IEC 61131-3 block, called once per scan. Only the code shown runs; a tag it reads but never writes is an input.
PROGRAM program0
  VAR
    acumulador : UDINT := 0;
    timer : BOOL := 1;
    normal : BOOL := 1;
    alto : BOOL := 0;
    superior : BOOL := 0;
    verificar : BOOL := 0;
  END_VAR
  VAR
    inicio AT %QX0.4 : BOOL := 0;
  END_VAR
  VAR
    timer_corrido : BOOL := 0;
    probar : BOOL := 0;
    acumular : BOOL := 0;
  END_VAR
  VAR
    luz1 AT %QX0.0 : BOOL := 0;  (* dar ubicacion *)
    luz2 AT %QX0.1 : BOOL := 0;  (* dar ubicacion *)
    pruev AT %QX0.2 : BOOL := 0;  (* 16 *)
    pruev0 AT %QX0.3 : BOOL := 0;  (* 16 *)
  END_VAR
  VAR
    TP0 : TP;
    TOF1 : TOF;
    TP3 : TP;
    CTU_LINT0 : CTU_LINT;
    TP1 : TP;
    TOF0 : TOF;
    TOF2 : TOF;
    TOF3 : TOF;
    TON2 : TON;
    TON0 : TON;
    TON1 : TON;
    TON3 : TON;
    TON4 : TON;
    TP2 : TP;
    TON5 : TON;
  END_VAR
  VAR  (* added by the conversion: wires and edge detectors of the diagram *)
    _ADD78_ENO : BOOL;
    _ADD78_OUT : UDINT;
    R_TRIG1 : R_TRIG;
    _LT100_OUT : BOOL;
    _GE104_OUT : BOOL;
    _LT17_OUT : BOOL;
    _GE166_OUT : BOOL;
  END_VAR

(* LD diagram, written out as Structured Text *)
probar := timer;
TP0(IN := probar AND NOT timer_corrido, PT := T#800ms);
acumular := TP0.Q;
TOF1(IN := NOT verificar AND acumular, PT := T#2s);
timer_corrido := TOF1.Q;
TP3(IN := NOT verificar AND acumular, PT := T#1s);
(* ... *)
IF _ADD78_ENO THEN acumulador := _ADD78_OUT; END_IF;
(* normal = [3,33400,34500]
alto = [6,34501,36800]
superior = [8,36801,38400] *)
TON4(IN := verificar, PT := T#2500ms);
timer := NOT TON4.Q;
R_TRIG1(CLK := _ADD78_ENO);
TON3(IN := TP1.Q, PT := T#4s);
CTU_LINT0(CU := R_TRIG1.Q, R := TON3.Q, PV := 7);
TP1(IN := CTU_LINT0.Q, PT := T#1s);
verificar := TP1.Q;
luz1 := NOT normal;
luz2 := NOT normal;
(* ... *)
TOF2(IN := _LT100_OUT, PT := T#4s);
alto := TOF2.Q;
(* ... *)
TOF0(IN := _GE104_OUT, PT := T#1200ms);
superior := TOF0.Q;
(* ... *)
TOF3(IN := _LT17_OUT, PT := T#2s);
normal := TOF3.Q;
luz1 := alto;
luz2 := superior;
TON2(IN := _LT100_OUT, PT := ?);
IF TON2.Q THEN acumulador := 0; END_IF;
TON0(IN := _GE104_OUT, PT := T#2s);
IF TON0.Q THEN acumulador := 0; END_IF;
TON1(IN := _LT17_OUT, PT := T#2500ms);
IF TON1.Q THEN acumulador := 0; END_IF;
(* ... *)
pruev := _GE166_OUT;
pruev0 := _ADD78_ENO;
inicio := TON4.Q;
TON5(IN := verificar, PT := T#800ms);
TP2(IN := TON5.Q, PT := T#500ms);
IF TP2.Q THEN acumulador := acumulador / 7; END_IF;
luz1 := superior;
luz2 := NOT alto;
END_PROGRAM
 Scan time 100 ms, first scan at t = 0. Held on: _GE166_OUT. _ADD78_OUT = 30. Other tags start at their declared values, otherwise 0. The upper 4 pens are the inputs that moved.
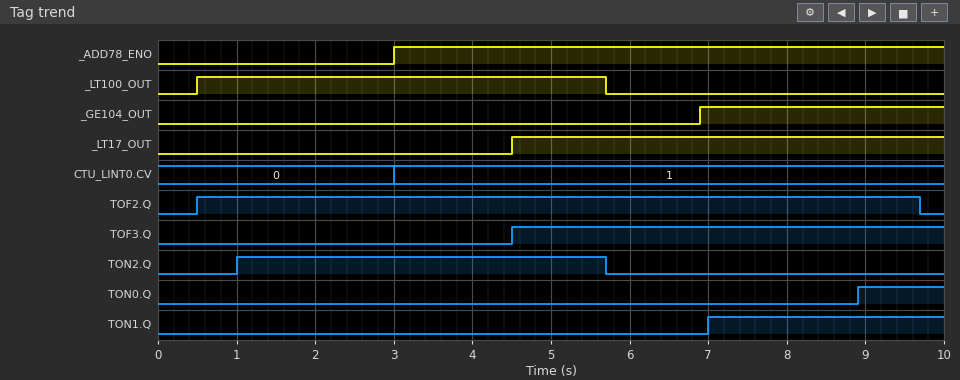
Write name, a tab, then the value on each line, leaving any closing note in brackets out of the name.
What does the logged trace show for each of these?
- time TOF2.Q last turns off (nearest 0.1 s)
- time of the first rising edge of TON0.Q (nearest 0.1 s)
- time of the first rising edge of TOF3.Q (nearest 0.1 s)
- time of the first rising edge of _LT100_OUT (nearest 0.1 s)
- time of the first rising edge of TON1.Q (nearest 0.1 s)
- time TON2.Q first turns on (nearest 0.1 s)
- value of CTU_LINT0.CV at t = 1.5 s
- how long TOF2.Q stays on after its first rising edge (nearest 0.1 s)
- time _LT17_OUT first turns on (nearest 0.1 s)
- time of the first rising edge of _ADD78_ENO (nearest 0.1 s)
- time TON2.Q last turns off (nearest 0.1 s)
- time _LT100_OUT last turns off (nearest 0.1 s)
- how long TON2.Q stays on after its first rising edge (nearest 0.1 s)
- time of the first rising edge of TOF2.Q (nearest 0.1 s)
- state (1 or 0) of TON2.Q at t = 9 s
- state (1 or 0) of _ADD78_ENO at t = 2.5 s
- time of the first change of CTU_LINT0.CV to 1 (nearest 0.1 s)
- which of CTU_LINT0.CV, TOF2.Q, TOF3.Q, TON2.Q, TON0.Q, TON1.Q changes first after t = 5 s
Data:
time TOF2.Q last turns off	9.7 s
time of the first rising edge of TON0.Q	8.9 s
time of the first rising edge of TOF3.Q	4.5 s
time of the first rising edge of _LT100_OUT	0.5 s
time of the first rising edge of TON1.Q	7.0 s
time TON2.Q first turns on	1.0 s
value of CTU_LINT0.CV at t = 1.5 s	0
how long TOF2.Q stays on after its first rising edge	9.2 s
time _LT17_OUT first turns on	4.5 s
time of the first rising edge of _ADD78_ENO	3.0 s
time TON2.Q last turns off	5.7 s
time _LT100_OUT last turns off	5.7 s
how long TON2.Q stays on after its first rising edge	4.7 s
time of the first rising edge of TOF2.Q	0.5 s
state (1 or 0) of TON2.Q at t = 9 s	0
state (1 or 0) of _ADD78_ENO at t = 2.5 s	0
time of the first change of CTU_LINT0.CV to 1	3.0 s
which of CTU_LINT0.CV, TOF2.Q, TOF3.Q, TON2.Q, TON0.Q, TON1.Q changes first after t = 5 s	TON2.Q
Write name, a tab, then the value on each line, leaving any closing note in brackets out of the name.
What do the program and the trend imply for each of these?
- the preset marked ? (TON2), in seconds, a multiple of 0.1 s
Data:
the preset marked ? (TON2), in seconds, a multiple of 0.1 s	0.5 s
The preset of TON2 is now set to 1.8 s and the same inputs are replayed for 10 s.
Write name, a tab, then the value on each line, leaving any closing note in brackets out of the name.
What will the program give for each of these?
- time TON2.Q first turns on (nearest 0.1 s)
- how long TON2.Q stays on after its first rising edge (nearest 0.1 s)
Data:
time TON2.Q first turns on	2.3 s
how long TON2.Q stays on after its first rising edge	3.4 s
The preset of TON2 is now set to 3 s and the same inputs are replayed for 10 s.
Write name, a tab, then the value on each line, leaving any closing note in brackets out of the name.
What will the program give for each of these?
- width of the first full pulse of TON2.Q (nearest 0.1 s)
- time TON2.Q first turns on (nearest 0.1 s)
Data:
width of the first full pulse of TON2.Q	2.2 s
time TON2.Q first turns on	3.5 s
